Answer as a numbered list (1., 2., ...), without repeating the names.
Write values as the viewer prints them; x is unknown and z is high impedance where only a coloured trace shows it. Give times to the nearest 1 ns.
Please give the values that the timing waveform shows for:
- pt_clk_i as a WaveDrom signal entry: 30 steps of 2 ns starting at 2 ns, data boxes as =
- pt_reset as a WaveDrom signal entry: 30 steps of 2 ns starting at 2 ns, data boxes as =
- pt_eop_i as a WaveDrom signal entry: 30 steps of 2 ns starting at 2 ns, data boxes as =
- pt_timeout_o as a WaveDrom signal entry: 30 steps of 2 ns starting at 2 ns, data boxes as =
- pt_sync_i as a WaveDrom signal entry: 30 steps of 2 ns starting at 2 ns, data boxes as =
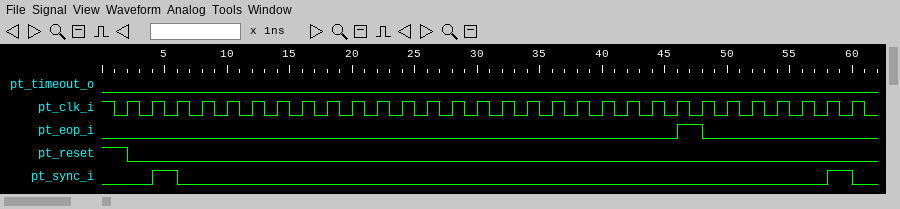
1. {name: 'pt_clk_i', wave: 'p.............................'}
2. {name: 'pt_reset', wave: '0.............................'}
3. {name: 'pt_eop_i', wave: '0.....................10......'}
4. {name: 'pt_timeout_o', wave: '0.............................'}
5. {name: 'pt_sync_i', wave: '010.........................10'}
